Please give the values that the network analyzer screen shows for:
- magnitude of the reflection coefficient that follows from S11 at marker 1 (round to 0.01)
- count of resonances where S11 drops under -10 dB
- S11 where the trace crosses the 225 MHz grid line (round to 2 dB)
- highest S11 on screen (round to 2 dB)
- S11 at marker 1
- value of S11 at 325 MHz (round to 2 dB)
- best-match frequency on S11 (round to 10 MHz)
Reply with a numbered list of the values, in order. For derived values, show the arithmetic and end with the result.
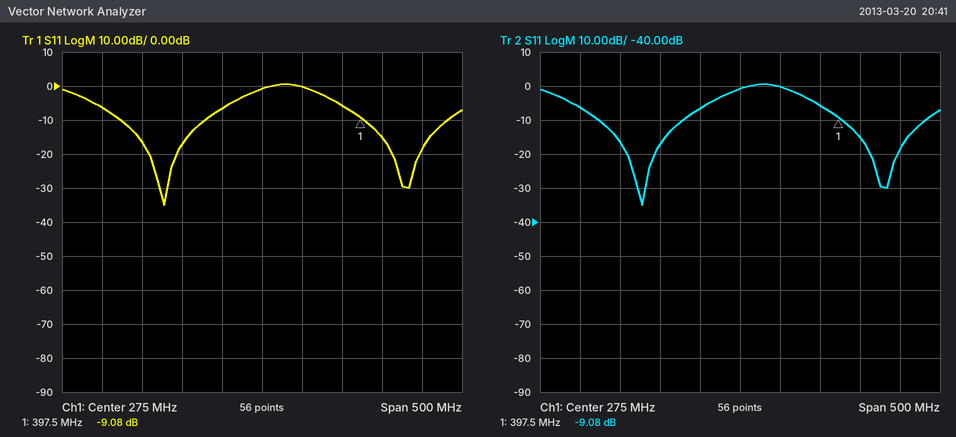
1. 10^(-9.08/20) ≈ 0.35
2. 2
3. -6 dB
4. 0 dB
5. -9.08 dB
6. 0 dB
7. 150 MHz
